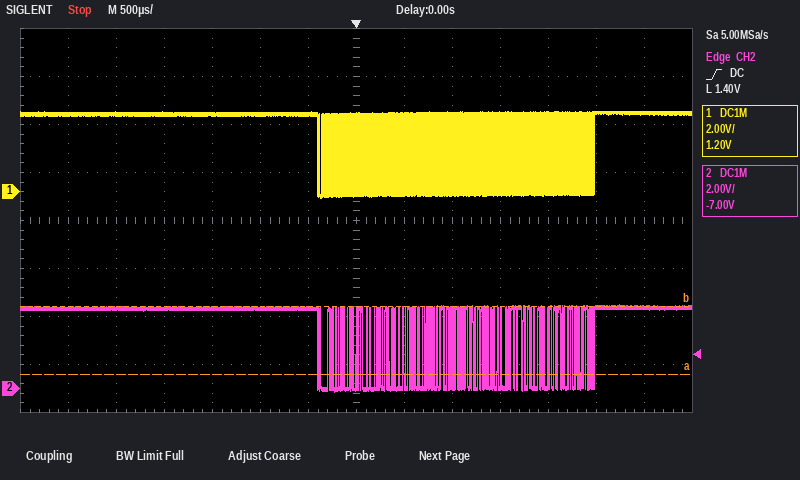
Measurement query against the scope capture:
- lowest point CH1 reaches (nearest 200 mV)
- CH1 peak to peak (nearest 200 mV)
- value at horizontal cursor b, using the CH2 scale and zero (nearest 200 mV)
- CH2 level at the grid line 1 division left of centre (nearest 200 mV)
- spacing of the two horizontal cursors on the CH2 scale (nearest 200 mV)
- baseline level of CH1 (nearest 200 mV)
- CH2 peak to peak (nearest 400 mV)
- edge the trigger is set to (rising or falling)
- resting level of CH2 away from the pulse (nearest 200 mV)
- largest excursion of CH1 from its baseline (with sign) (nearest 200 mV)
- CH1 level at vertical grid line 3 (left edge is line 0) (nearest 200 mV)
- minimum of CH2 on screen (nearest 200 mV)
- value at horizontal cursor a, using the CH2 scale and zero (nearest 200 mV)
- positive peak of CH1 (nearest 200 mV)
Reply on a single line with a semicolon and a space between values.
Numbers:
-200 mV; 3.6 V; 3.4 V; 3.4 V; 2.8 V; 3.2 V; 3.6 V; rising; 3.4 V; -3.4 V; 3.2 V; -200 mV; 600 mV; 3.4 V
